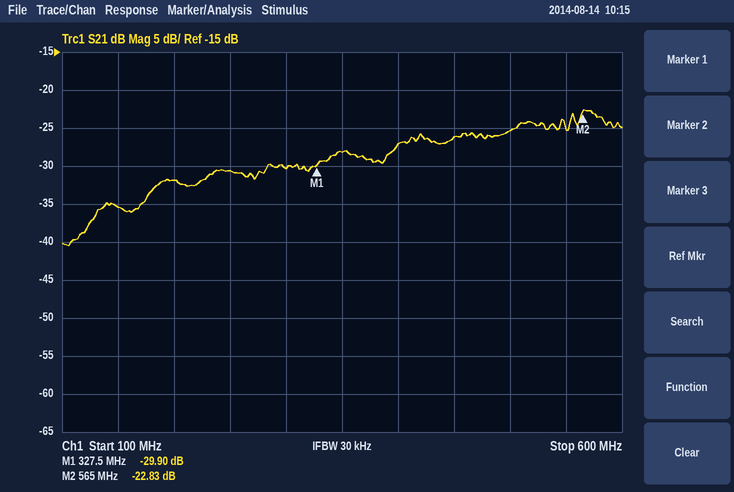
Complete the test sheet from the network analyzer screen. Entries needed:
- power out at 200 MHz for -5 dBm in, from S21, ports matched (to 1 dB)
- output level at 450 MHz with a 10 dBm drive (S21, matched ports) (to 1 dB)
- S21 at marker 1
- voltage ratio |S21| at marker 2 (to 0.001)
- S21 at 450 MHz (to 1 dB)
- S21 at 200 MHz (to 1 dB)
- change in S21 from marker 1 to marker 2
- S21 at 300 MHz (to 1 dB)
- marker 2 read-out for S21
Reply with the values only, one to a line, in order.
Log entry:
-37 dBm
-16 dBm
-29.90 dB
0.072
-26 dB
-32 dB
7.07 dB
-30 dB
-22.83 dB
